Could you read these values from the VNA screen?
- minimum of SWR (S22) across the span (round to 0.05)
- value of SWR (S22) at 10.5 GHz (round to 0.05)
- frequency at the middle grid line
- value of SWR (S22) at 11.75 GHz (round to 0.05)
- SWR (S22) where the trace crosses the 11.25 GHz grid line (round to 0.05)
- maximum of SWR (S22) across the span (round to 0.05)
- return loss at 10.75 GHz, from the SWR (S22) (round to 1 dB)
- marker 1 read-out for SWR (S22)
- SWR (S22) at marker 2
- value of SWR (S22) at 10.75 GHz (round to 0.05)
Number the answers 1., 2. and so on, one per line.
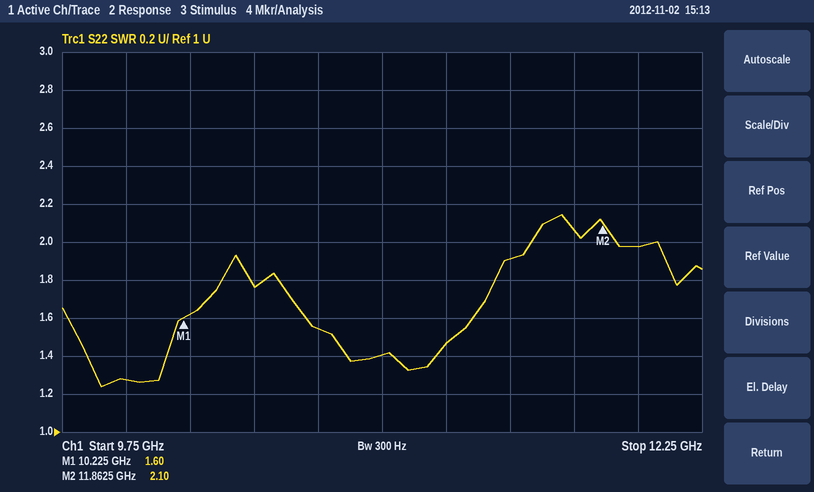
1. 1.25
2. 1.75
3. 11 GHz
4. 2.05
5. 1.45
6. 2.15
7. 13 dB
8. 1.60
9. 2.10
10. 1.55
